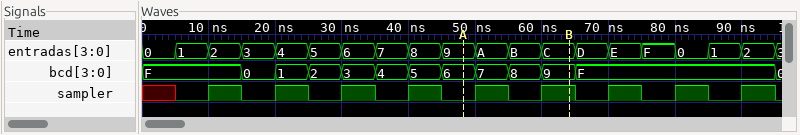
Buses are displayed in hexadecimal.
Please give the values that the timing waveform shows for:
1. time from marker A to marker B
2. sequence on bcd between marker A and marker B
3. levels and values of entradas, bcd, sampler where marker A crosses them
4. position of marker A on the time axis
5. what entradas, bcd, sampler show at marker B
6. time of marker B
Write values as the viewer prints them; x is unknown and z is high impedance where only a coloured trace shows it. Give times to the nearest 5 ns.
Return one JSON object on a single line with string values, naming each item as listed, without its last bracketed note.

{"time from marker A to marker B": "15 ns", "sequence on bcd between marker A and marker B": "6, 7, 8, 9", "levels and values of entradas, bcd, sampler where marker A crosses them": "entradas=9, bcd=6, sampler=0", "position of marker A on the time axis": "50 ns", "what entradas, bcd, sampler show at marker B": "entradas=C, bcd=9, sampler=1", "time of marker B": "65 ns"}
